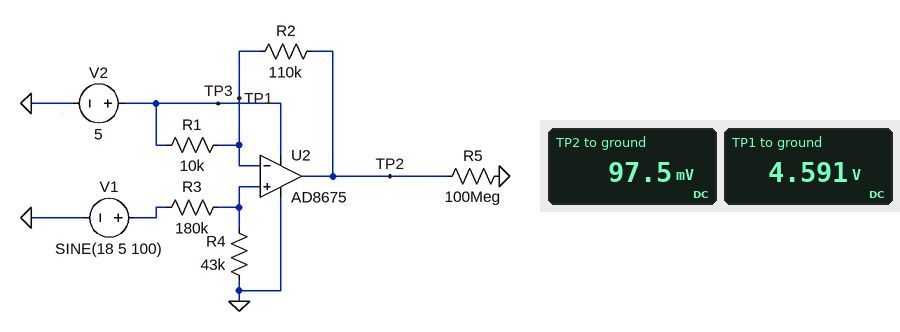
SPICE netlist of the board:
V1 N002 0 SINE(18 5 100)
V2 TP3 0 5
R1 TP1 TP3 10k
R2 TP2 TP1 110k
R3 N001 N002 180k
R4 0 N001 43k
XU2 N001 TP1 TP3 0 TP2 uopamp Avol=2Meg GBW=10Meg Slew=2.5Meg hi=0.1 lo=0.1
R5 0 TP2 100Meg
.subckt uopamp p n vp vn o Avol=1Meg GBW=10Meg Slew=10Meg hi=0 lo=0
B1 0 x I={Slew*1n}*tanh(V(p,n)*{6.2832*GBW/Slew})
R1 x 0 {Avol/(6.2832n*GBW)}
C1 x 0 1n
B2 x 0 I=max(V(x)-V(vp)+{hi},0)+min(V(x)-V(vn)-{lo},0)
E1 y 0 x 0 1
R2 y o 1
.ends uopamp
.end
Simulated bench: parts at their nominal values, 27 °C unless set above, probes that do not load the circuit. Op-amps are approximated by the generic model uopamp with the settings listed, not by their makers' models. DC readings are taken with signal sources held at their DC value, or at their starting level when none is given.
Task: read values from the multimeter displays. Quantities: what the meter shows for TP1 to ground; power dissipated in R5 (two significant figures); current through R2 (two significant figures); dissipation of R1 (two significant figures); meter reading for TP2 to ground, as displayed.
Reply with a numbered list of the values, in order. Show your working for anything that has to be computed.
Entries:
1. 4.591 V
2. (97.5 mV)^2 / 100 MΩ = 95 pW
3. (4.591 V - 97.5 mV) / 110 kΩ = 41 µA
4. (5 V - 4.591 V)^2 / 10 kΩ = 17 µW
5. 97.5 mV
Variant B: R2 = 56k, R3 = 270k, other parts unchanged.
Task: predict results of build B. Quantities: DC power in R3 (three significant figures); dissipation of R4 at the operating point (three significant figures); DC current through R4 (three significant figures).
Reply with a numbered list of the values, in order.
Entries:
1. 893 µW
2. 142 µW
3. 57.5 µA
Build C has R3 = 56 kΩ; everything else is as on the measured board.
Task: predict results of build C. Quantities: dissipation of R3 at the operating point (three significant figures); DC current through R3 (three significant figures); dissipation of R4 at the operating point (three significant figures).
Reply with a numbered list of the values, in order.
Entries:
1. 1.85 mW
2. 182 µA
3. 1.42 mW
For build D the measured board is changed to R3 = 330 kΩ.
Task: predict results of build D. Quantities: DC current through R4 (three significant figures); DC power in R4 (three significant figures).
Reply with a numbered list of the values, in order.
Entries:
1. 48.3 µA
2. 100 µW
